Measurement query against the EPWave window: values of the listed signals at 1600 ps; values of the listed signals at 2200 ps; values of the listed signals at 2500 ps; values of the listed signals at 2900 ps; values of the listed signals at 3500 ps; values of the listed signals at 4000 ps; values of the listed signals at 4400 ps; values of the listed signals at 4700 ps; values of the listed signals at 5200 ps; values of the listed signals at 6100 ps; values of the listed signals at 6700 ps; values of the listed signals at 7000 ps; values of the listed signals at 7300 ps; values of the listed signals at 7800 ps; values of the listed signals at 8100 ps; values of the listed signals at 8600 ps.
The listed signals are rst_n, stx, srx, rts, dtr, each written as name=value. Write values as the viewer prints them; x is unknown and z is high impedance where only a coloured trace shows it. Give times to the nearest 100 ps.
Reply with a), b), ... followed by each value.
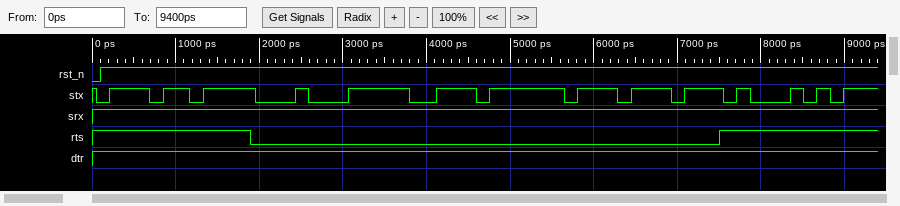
a) rst_n=1, stx=1, srx=1, rts=1, dtr=1
b) rst_n=1, stx=0, srx=1, rts=0, dtr=1
c) rst_n=1, stx=1, srx=1, rts=0, dtr=1
d) rst_n=1, stx=0, srx=1, rts=0, dtr=1
e) rst_n=1, stx=1, srx=1, rts=0, dtr=1
f) rst_n=1, stx=0, srx=1, rts=0, dtr=1
g) rst_n=1, stx=1, srx=1, rts=0, dtr=1
h) rst_n=1, stx=0, srx=1, rts=0, dtr=1
i) rst_n=1, stx=1, srx=1, rts=0, dtr=1
j) rst_n=1, stx=1, srx=1, rts=0, dtr=1
k) rst_n=1, stx=1, srx=1, rts=0, dtr=1
l) rst_n=1, stx=0, srx=1, rts=0, dtr=1
m) rst_n=1, stx=1, srx=1, rts=0, dtr=1
n) rst_n=1, stx=1, srx=1, rts=1, dtr=1
o) rst_n=1, stx=0, srx=1, rts=1, dtr=1
p) rst_n=1, stx=0, srx=1, rts=1, dtr=1
